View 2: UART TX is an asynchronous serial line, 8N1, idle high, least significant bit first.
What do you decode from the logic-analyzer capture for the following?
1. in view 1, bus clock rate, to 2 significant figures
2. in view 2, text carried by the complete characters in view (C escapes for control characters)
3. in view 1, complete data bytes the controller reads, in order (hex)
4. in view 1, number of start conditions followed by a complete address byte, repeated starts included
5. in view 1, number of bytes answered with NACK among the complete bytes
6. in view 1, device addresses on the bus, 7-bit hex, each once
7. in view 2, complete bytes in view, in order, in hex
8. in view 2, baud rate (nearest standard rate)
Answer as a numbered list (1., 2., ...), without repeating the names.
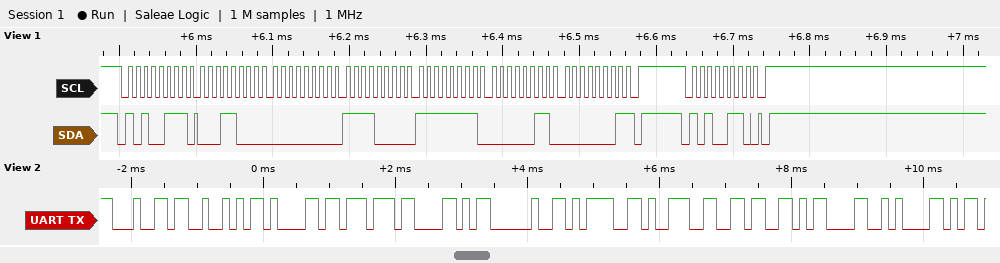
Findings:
1. 100 kHz
2. "dRawX =96\r\n"
3. 18 00 F0 FF 03 01
4. 2
5. 1
6. 0x53
7. 64 52 61 77 58 20 3D 39 36 0D 0A
8. 9600 baud
